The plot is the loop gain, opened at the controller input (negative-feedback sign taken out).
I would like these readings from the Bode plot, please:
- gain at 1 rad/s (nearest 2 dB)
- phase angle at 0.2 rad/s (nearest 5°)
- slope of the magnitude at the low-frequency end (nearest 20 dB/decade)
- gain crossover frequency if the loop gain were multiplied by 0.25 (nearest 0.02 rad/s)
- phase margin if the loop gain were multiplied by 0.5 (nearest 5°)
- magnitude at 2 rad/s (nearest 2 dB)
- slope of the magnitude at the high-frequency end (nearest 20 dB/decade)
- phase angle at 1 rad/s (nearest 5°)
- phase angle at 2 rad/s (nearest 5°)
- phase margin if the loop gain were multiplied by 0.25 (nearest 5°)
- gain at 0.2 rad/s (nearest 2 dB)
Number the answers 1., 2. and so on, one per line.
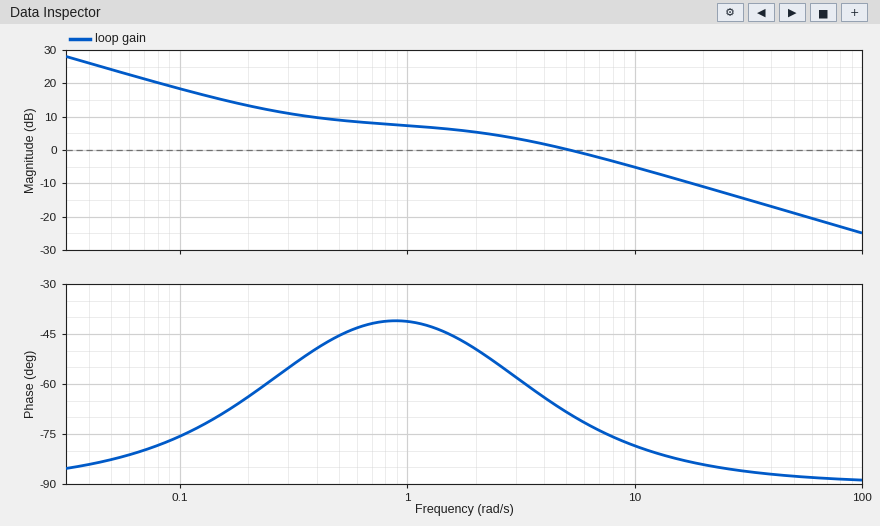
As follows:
1. 8 dB
2. -65°
3. -20 dB/decade
4. 0.24 rad/s
5. 135°
6. 6 dB
7. -20 dB/decade
8. -40°
9. -50°
10. 120°
11. 14 dB
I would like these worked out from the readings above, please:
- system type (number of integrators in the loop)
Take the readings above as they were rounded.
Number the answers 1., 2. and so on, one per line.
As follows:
1. 1
